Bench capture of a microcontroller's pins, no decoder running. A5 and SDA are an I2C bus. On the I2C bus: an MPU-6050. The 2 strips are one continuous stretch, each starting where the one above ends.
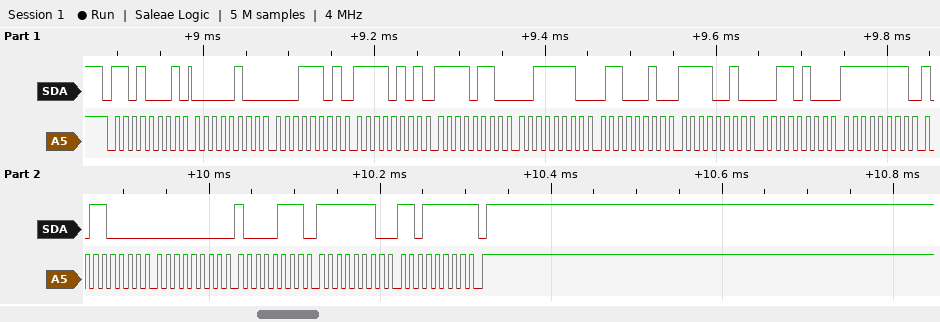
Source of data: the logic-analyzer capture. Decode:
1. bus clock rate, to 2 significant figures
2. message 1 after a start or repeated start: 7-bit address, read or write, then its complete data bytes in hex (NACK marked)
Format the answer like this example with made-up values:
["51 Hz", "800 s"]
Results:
["100 kHz", "0x68 read: 04 1D F5 F6 3E 62 F2 34 FF B0 00 87 FE DF NACK"]
